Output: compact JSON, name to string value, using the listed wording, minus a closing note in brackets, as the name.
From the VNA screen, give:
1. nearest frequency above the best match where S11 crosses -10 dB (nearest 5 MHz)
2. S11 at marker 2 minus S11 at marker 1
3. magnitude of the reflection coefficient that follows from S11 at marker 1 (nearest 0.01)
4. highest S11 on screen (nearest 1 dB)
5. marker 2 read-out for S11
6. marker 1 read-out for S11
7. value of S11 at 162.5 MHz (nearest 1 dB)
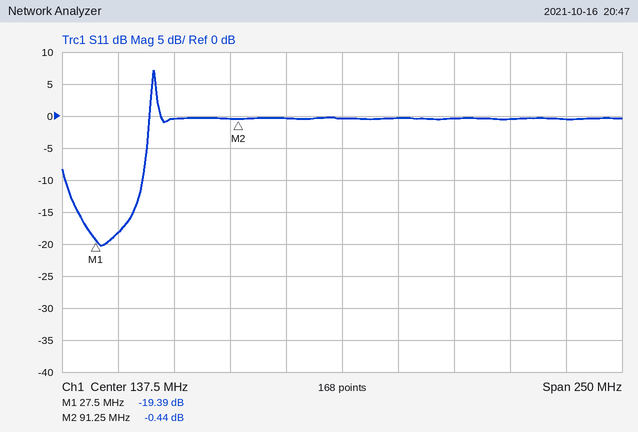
{"nearest frequency above the best match where S11 crosses -10 dB": "50 MHz", "S11 at marker 2 minus S11 at marker 1": "18.95 dB", "magnitude of the reflection coefficient that follows from S11 at marker 1": "0.11", "highest S11 on screen": "7 dB", "marker 2 read-out for S11": "-0.44 dB", "marker 1 read-out for S11": "-19.39 dB", "value of S11 at 162.5 MHz": "0 dB"}
